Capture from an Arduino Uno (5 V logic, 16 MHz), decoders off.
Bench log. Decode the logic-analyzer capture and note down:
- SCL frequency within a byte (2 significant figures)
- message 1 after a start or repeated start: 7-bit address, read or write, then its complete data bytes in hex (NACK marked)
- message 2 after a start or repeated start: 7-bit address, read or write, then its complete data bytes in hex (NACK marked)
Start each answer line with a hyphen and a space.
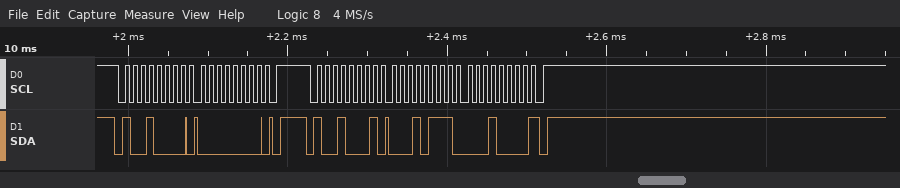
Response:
- 100 kHz
- 0x48 write: 00
- 0x48 read: 17 10 NACK
